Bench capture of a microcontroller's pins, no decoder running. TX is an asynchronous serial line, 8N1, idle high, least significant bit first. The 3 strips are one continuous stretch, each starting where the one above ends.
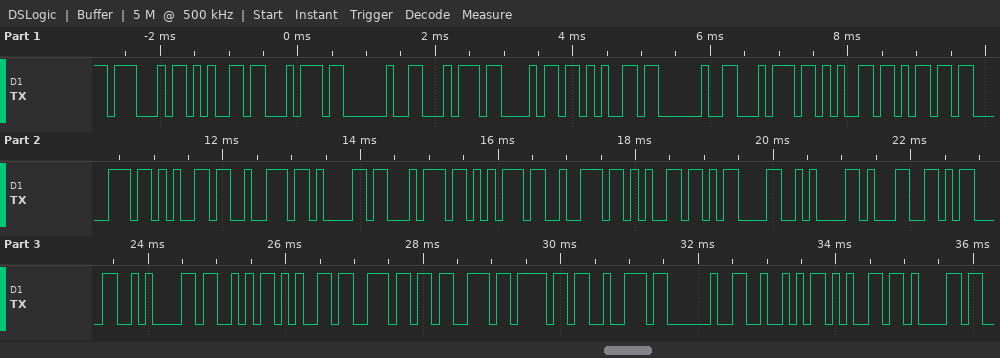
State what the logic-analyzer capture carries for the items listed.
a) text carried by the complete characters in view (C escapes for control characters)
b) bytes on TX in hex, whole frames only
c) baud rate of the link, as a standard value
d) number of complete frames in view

"Get the temperature\r\n1\r\nSensor Rea"
47 65 74 20 74 68 65 20 74 65 6D 70 65 72 61 74 75 72 65 0D 0A 31 0D 0A 53 65 6E 73 6F 72 20 52 65 61
9600 baud
34
